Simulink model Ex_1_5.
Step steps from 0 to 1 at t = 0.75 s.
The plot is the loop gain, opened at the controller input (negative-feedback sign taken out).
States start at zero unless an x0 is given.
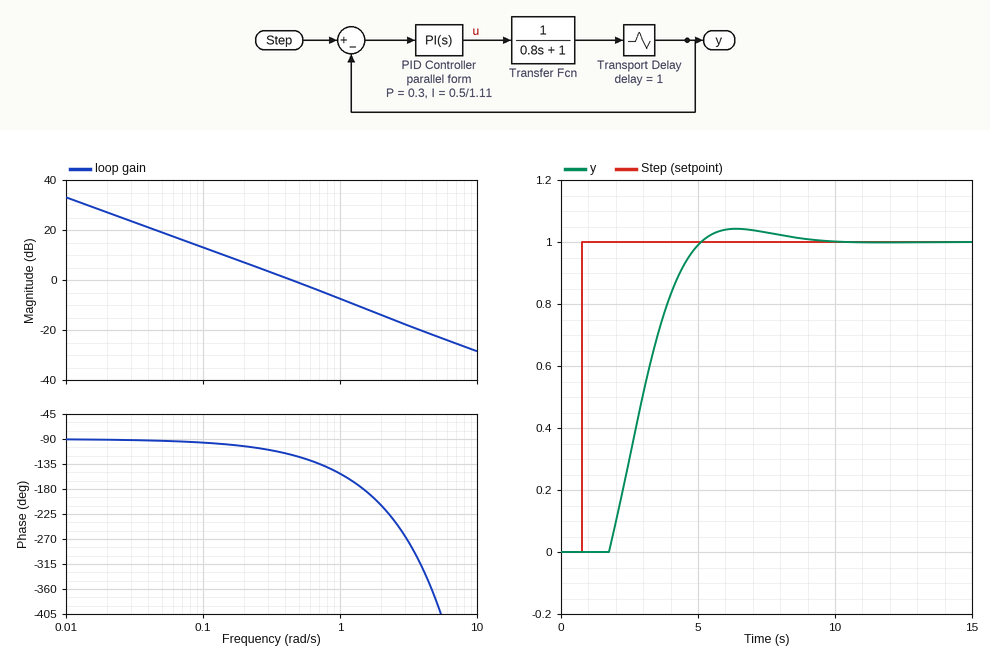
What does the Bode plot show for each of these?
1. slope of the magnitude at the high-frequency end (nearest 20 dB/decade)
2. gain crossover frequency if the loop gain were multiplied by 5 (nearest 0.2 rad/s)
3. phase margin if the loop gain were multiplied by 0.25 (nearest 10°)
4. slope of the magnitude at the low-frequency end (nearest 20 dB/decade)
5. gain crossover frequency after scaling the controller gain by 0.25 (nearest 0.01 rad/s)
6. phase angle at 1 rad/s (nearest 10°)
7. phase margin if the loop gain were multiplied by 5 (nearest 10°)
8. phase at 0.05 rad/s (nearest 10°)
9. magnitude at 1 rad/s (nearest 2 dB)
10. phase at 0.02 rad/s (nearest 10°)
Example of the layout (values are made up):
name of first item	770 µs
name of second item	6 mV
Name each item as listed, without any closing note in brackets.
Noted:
slope of the magnitude at the high-frequency end	-20 dB/decade
gain crossover frequency if the loop gain were multiplied by 5	2.0 rad/s
phase margin if the loop gain were multiplied by 0.25	80°
slope of the magnitude at the low-frequency end	-20 dB/decade
gain crossover frequency after scaling the controller gain by 0.25	0.11 rad/s
phase angle at 1 rad/s	-150°
phase margin if the loop gain were multiplied by 5	-30°
phase at 0.05 rad/s	-90°
magnitude at 1 rad/s	-8 dB
phase at 0.02 rad/s	-90°
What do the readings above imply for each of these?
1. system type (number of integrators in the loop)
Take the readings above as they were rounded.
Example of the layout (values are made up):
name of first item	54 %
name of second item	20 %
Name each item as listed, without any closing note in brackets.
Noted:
system type	1
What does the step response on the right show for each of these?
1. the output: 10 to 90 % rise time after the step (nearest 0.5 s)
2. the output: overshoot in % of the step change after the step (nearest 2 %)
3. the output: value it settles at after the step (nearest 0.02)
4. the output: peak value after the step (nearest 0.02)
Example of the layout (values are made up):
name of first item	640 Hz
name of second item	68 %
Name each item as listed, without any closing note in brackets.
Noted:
the output: 10 to 90 % rise time after the step	2.5 s
the output: overshoot in % of the step change after the step	4 %
the output: value it settles at after the step	1.00
the output: peak value after the step	1.04
